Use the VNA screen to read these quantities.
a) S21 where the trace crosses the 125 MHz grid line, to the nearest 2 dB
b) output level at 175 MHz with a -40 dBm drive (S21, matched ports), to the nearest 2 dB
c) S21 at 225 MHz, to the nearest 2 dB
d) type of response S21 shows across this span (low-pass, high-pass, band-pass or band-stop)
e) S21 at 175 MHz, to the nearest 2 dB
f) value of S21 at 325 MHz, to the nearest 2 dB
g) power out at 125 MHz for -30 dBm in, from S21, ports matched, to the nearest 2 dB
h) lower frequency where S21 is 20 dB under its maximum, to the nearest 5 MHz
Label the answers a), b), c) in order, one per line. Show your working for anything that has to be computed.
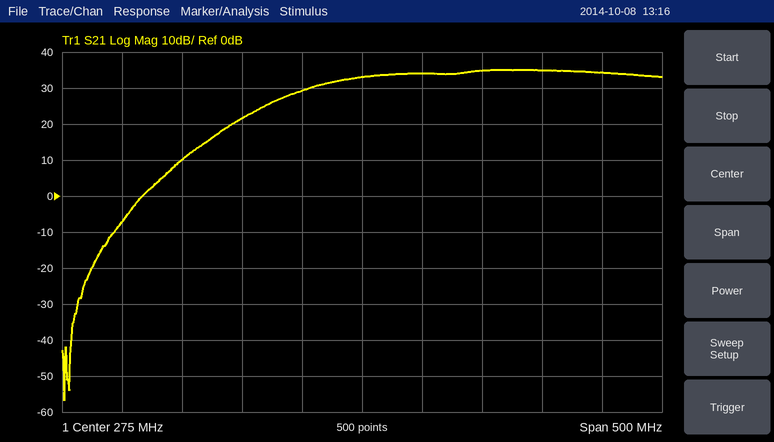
a) 10 dB
b) -40 dBm + (22 dB) = -18 dBm
c) 30 dB
d) high-pass
e) 22 dB
f) 34 dB
g) -30 dBm + (10 dB) = -20 dBm
h) 145 MHz
